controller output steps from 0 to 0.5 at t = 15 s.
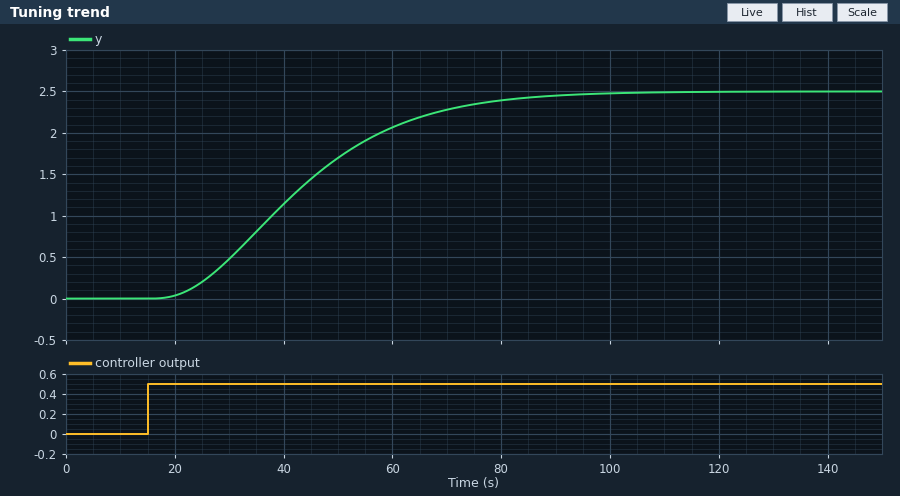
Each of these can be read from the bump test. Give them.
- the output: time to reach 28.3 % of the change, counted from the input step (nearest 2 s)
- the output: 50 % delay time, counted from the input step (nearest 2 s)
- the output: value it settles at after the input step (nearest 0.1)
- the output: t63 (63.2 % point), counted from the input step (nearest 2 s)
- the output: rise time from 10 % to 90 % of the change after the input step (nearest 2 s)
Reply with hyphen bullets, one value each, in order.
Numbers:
- 18 s
- 26 s
- 2.5
- 32 s
- 42 s
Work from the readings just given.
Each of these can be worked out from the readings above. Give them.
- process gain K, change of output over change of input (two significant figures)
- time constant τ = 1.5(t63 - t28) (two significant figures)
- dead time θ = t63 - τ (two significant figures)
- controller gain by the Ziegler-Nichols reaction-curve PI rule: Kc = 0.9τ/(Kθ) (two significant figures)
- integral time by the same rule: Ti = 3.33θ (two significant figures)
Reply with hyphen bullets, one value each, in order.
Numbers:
- 5.0
- 21 s
- 11 s
- 0.34
- 37 s
